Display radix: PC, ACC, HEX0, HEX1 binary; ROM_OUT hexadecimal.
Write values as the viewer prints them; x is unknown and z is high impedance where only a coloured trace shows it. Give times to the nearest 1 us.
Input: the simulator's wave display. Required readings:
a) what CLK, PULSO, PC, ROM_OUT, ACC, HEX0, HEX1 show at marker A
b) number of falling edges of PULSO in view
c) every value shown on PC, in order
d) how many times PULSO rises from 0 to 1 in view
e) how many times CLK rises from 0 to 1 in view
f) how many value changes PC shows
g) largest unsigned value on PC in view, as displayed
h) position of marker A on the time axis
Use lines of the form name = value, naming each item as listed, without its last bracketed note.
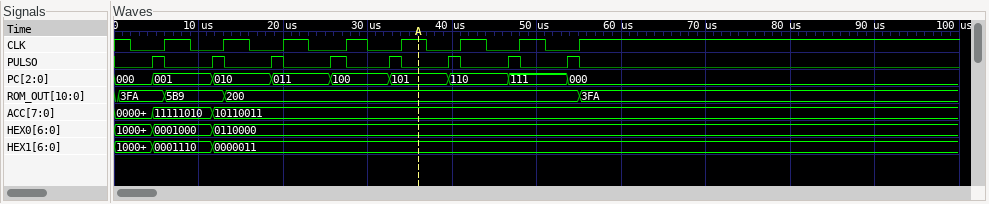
what CLK, PULSO, PC, ROM_OUT, ACC, HEX0, HEX1 show at marker A = CLK=1, PULSO=0, PC=101, ROM_OUT=200, ACC=10110011, HEX0=0110000, HEX1=0000011
number of falling edges of PULSO in view = 8
every value shown on PC, in order = 000, 001, 010, 011, 100, 101, 110, 111, 000
how many times PULSO rises from 0 to 1 in view = 8
how many times CLK rises from 0 to 1 in view = 8
how many value changes PC shows = 8
largest unsigned value on PC in view, as displayed = 111
position of marker A on the time axis = 36 us
